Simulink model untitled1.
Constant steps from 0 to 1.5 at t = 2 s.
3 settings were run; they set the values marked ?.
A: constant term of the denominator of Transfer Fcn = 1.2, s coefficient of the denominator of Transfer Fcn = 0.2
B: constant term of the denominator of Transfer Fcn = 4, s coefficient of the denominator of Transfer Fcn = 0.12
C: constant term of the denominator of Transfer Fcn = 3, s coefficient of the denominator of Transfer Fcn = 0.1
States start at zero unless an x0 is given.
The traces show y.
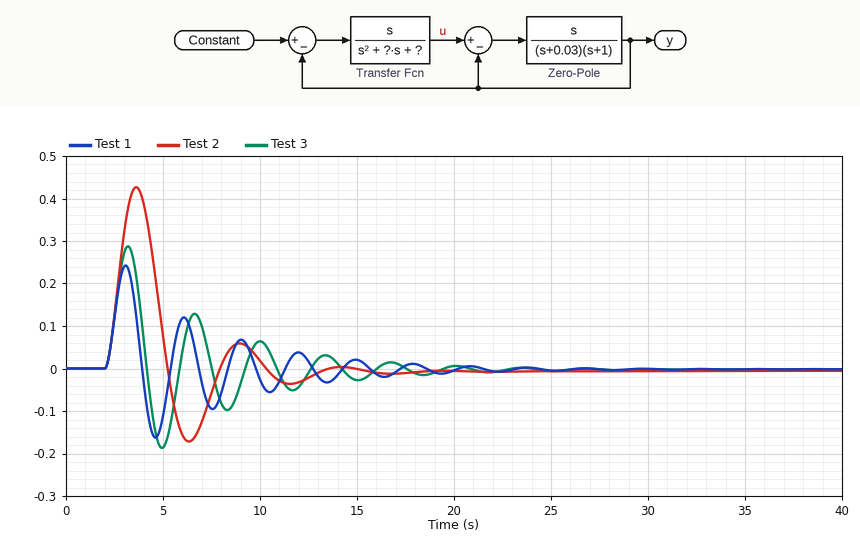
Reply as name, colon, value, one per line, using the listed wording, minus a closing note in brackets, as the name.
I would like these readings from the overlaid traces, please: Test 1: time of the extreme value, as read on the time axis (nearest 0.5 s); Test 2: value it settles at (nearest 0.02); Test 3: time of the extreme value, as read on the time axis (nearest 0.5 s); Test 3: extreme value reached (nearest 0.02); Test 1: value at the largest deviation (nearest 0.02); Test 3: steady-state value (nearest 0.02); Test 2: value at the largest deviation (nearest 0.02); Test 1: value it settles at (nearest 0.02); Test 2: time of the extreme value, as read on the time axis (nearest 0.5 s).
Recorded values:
Test 1: time of the extreme value, as read on the time axis: 3.0 s
Test 2: value it settles at: 0.00
Test 3: time of the extreme value, as read on the time axis: 3.0 s
Test 3: extreme value reached: 0.28
Test 1: value at the largest deviation: 0.24
Test 3: steady-state value: 0.00
Test 2: value at the largest deviation: 0.42
Test 1: value it settles at: 0.00
Test 2: time of the extreme value, as read on the time axis: 3.5 s
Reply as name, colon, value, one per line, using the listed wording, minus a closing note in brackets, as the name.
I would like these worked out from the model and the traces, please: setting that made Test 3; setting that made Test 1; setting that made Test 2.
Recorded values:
setting that made Test 3: C
setting that made Test 1: B
setting that made Test 2: A
